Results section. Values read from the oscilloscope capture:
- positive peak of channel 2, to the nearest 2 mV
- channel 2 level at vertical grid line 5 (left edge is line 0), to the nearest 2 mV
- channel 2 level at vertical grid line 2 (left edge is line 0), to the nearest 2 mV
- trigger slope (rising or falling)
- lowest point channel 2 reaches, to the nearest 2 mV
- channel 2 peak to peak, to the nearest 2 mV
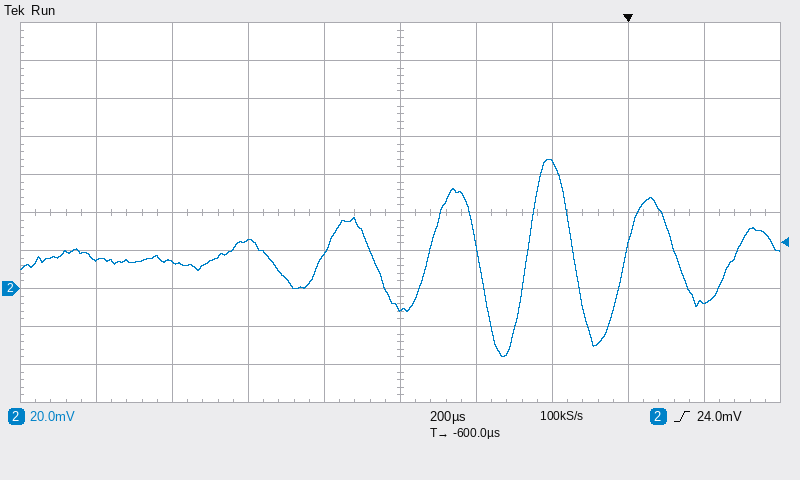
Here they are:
68 mV
-10 mV
14 mV
rising
-36 mV
104 mV
